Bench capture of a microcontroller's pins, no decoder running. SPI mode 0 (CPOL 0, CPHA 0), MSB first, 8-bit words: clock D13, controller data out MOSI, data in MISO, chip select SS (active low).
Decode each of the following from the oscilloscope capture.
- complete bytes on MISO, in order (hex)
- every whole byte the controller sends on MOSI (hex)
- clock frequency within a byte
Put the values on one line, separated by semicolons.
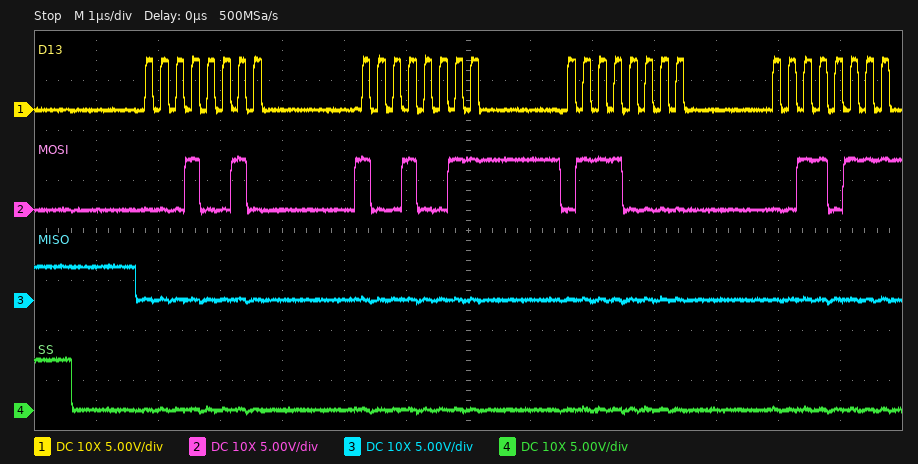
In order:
0x00 0x00 0x00 0x00; 0x12 0x93 0x70 0x37; 4 MHz
